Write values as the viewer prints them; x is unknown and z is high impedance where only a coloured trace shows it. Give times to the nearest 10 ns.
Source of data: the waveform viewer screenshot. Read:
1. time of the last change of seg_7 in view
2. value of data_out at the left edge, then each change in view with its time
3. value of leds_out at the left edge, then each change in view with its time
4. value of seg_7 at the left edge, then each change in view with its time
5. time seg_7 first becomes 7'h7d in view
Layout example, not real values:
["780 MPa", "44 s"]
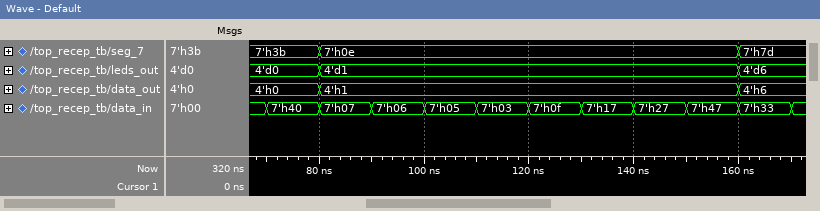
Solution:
["160 ns", "4'h0, 4'h1 at 80 ns, 4'h6 at 160 ns", "4'd0, 4'd1 at 80 ns, 4'd6 at 160 ns", "7'h3b, 7'h0e at 80 ns, 7'h7d at 160 ns", "160 ns"]
